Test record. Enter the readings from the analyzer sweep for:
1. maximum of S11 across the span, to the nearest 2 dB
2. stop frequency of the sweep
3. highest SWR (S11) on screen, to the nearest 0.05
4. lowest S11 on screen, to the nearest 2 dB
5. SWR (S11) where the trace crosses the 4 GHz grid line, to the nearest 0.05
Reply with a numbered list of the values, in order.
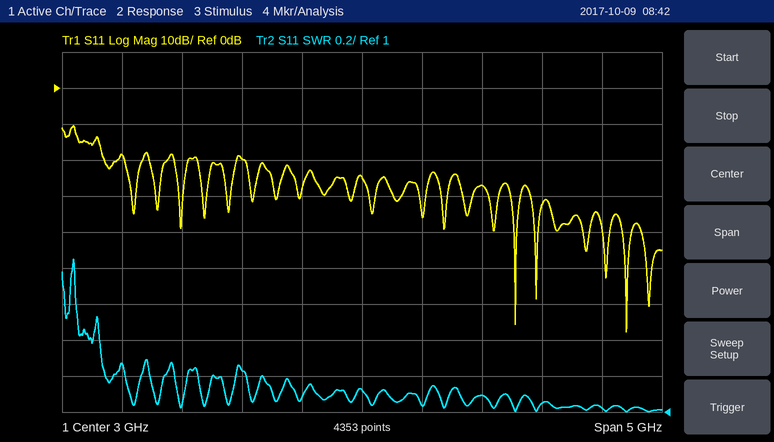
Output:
1. -10 dB
2. 5.5 GHz
3. 1.85
4. -68 dB
5. 1.10
